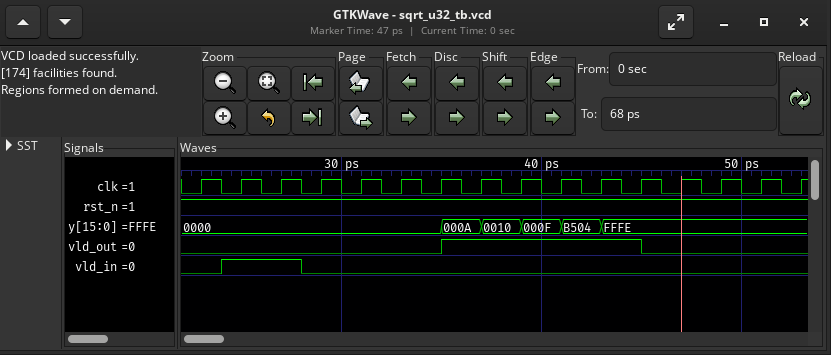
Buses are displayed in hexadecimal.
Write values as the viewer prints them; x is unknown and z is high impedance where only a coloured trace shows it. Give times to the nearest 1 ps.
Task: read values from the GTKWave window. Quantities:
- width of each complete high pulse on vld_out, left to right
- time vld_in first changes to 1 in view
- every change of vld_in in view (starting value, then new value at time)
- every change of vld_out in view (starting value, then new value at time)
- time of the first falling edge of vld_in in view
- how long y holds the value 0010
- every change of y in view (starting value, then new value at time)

10 ps
24 ps
0, 1 at 24 ps, 0 at 28 ps
0, 1 at 35 ps, 0 at 45 ps
28 ps
2 ps
0000, 000A at 35 ps, 0010 at 37 ps, 000F at 39 ps, B504 at 41 ps, FFFE at 43 ps
